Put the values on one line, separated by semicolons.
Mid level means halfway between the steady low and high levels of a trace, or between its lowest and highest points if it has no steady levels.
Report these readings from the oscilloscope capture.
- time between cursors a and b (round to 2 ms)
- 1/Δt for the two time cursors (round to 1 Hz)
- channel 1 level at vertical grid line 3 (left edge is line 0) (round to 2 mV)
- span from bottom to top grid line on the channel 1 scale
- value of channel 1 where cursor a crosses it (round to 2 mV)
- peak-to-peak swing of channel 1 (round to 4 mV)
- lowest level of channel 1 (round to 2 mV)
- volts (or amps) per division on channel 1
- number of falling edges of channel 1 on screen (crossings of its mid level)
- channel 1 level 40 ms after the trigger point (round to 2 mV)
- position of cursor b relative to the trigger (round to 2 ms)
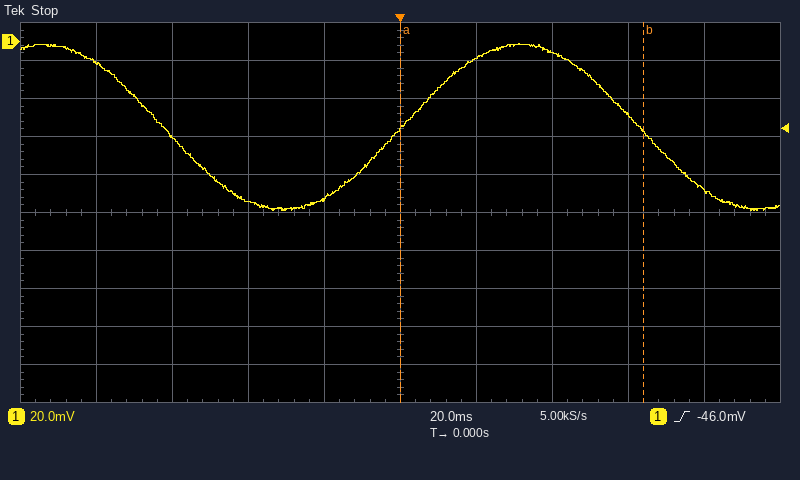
64 ms; 16 Hz; -84 mV; 200 mV; -46 mV; 88 mV; -88 mV; 20 mV; 2; -6 mV; +64 ms
